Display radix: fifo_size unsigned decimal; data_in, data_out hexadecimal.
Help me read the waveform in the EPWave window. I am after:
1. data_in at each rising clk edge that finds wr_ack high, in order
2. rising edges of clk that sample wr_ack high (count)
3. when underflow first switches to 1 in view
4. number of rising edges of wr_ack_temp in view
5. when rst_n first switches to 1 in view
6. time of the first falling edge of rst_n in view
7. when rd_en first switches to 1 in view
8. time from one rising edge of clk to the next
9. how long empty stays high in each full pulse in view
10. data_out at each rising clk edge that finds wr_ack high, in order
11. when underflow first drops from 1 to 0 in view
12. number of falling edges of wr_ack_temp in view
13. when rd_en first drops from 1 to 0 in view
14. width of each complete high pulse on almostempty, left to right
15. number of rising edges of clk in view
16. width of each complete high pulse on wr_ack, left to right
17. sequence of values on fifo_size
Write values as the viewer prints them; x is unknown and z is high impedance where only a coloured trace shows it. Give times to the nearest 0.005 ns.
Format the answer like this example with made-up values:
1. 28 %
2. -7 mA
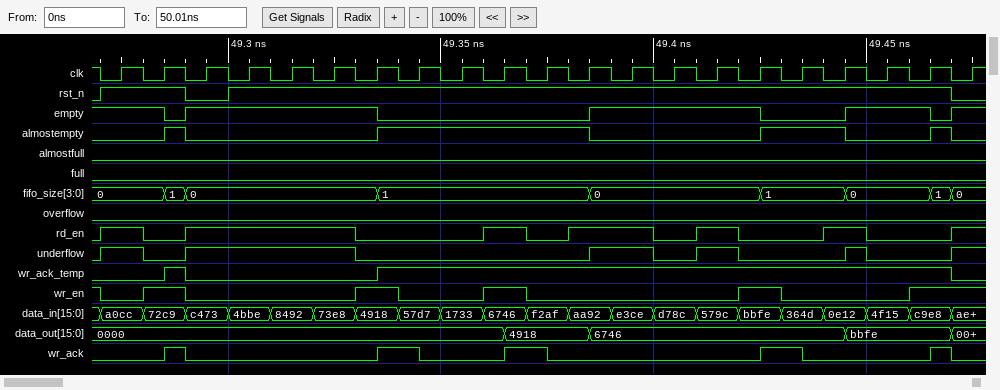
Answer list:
1. 57d7, f2af, 364d
2. 3
3. 49.27 ns
4. 2
5. 49.27 ns
6. 49.29 ns
7. 49.27 ns
8. 0.01 ns
9. 0.045 ns, 0.04 ns, 0.02 ns
10. 0000, 4918, 6746
11. 49.28 ns
12. 2
13. 49.28 ns
14. 0.005 ns, 0.05 ns, 0.02 ns, 0.005 ns
15. 21
16. 0.005 ns, 0.01 ns, 0.01 ns, 0.01 ns, 0.005 ns
17. 0, 1, 0, 1, 0, 1, 0, 1, 0
